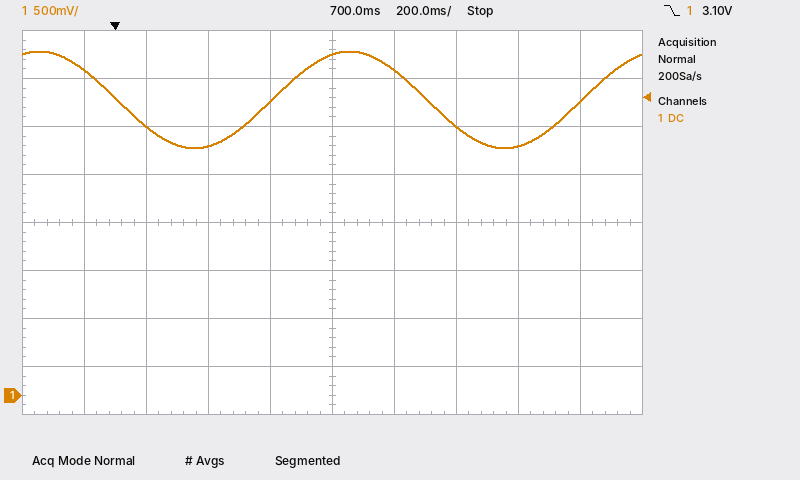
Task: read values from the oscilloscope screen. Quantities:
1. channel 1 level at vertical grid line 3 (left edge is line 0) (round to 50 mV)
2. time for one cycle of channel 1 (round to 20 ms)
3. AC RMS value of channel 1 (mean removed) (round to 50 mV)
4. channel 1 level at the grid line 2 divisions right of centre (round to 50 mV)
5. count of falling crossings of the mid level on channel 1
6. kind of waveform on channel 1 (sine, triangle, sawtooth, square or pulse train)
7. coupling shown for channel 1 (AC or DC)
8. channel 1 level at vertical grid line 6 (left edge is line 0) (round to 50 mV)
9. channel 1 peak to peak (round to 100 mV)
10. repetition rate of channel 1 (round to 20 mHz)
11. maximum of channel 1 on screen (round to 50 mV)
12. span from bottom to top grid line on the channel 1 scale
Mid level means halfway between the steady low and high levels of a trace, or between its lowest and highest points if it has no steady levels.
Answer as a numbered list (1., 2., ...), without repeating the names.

1. 2.60 V
2. 1.00 s
3. 350 mV
4. 2.80 V
5. 2
6. sine
7. DC
8. 3.40 V
9. 1.00 V
10. 1.00 Hz
11. 3.60 V
12. 4 V
